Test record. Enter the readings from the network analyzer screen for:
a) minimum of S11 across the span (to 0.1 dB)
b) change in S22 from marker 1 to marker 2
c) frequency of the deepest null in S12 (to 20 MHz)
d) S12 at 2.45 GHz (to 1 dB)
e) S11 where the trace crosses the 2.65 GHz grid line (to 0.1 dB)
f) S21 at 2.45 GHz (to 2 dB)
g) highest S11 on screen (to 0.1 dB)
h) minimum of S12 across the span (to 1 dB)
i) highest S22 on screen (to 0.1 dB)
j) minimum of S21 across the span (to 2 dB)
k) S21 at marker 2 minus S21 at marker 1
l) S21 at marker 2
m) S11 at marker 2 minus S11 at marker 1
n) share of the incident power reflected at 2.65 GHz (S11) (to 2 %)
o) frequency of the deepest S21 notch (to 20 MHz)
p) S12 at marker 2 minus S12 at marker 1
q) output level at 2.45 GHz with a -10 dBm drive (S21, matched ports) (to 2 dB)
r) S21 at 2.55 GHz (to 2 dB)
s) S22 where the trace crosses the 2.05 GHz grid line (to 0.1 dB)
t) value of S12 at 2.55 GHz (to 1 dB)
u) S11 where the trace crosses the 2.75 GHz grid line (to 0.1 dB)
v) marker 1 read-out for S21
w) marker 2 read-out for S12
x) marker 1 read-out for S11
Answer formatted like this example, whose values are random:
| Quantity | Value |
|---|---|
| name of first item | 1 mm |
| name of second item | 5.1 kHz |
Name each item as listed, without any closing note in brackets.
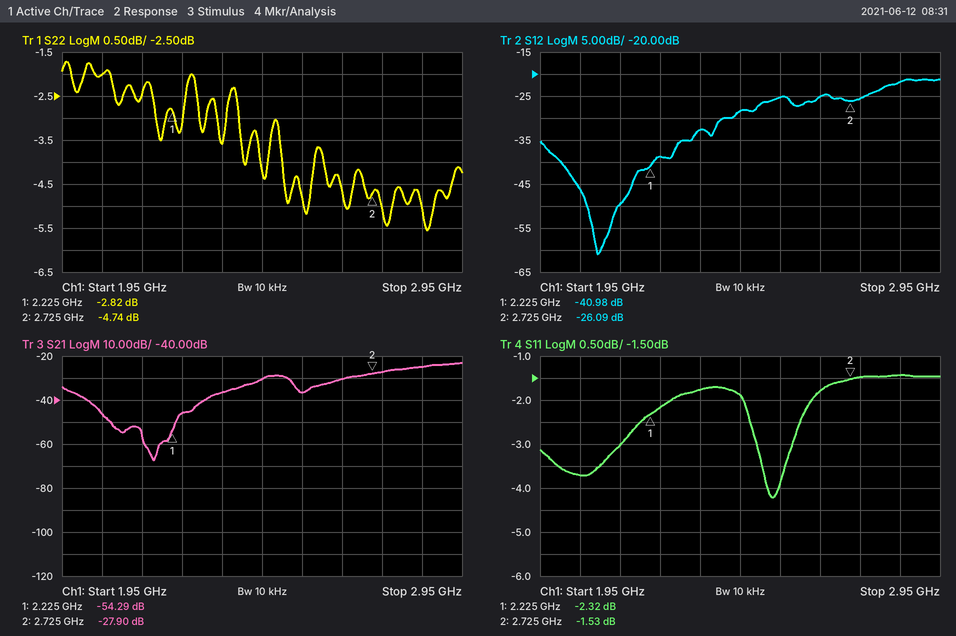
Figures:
| Quantity | Value |
|---|---|
| minimum of S11 across the span | -4.2 dB |
| change in S22 from marker 1 to marker 2 | -1.92 dB |
| frequency of the deepest null in S12 | 2.10 GHz |
| S12 at 2.45 GHz | -28 dB |
| S11 where the trace crosses the 2.65 GHz grid line | -1.8 dB |
| S21 at 2.45 GHz | -30 dB |
| highest S11 on screen | -1.4 dB |
| minimum of S12 across the span | -61 dB |
| highest S22 on screen | -1.7 dB |
| minimum of S21 across the span | -68 dB |
| S21 at marker 2 minus S21 at marker 1 | 26.39 dB |
| S21 at marker 2 | -27.90 dB |
| S11 at marker 2 minus S11 at marker 1 | 0.79 dB |
| share of the incident power reflected at 2.65 GHz (S11) | 66 % |
| frequency of the deepest S21 notch | 2.18 GHz |
| S12 at marker 2 minus S12 at marker 1 | 14.89 dB |
| output level at 2.45 GHz with a -10 dBm drive (S21, matched ports) | -40 dBm |
| S21 at 2.55 GHz | -36 dB |
| S22 where the trace crosses the 2.05 GHz grid line | -2.0 dB |
| value of S12 at 2.55 GHz | -25 dB |
| S11 where the trace crosses the 2.75 GHz grid line | -1.5 dB |
| marker 1 read-out for S21 | -54.29 dB |
| marker 2 read-out for S12 | -26.09 dB |
| marker 1 read-out for S11 | -2.32 dB |
